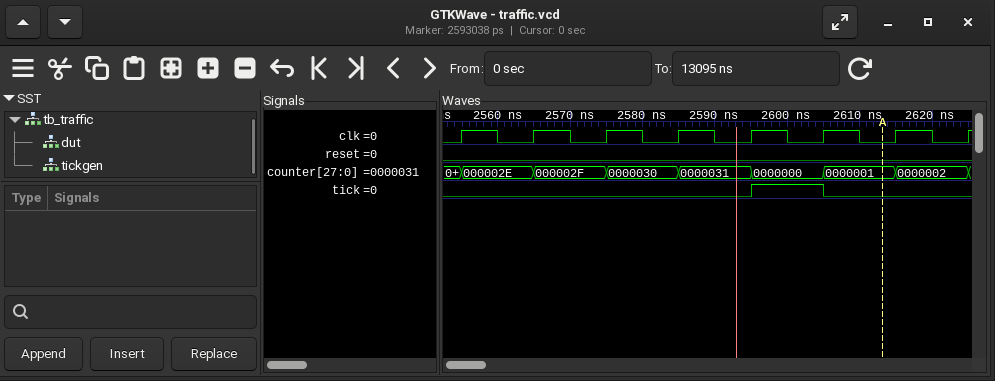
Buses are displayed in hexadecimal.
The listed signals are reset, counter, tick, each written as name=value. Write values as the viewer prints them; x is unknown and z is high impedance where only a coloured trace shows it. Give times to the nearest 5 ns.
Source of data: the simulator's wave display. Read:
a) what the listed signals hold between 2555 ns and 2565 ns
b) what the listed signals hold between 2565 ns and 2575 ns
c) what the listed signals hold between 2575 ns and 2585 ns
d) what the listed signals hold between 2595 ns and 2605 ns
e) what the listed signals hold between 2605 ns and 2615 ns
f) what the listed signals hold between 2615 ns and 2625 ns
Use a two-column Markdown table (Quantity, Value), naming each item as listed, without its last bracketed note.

| Quantity | Value |
|---|---|
| what the listed signals hold between 2555 ns and 2565 ns | reset=0, counter=000002E, tick=0 |
| what the listed signals hold between 2565 ns and 2575 ns | reset=0, counter=000002F, tick=0 |
| what the listed signals hold between 2575 ns and 2585 ns | reset=0, counter=0000030, tick=0 |
| what the listed signals hold between 2595 ns and 2605 ns | reset=0, counter=0000000, tick=1 |
| what the listed signals hold between 2605 ns and 2615 ns | reset=0, counter=0000001, tick=0 |
| what the listed signals hold between 2615 ns and 2625 ns | reset=0, counter=0000002, tick=0 |
